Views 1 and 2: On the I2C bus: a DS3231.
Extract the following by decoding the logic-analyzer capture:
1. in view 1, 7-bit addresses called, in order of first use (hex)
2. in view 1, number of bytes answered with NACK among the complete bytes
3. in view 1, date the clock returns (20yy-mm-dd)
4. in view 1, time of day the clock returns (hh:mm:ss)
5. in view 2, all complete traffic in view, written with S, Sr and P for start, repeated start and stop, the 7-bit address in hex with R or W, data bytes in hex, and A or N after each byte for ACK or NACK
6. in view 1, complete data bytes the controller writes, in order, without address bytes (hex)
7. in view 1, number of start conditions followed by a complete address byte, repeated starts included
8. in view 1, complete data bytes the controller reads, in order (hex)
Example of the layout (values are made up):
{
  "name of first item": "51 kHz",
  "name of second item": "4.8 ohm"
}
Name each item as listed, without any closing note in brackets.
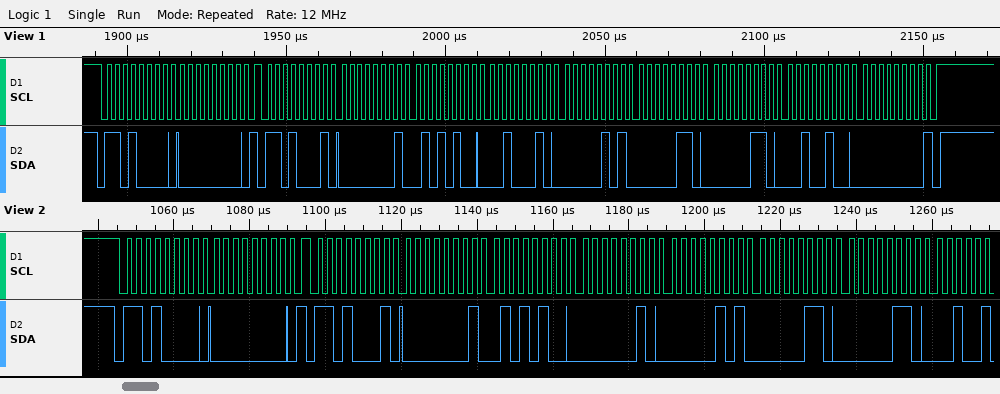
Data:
{
  "in view 1, 7-bit addresses called, in order of first use": "0x68",
  "in view 1, number of bytes answered with NACK among the complete bytes": "1",
  "in view 1, date the clock returns": "2024-06-06",
  "in view 1, time of day the clock returns": "22:54:01",
  "in view 2, all complete traffic in view, written with S, Sr and P for start, repeated start and stop, the 7-bit address in hex with R or W, data bytes in hex, and A or N after each byte for ACK or NACK": "S 68W A 00 A Sr 68R A 01 A 54 A 02 A 05 A 06 A 06 A",
  "in view 1, complete data bytes the controller writes, in order, without address bytes": "00",
  "in view 1, number of start conditions followed by a complete address byte, repeated starts included": "2",
  "in view 1, complete data bytes the controller reads, in order": "01 54 22 05 06 06 24 00"
}
